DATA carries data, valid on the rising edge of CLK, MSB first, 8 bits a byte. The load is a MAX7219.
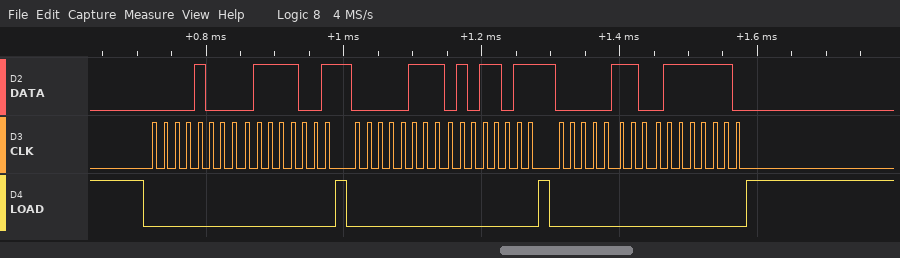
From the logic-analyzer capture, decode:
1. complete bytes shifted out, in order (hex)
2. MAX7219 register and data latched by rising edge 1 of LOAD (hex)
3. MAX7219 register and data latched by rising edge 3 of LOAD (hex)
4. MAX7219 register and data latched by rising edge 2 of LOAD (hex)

0x08 0x79 0x07 0x5B 0x06 0x7E
register 0x8, data 0x79
register 0x6, data 0x7E
register 0x7, data 0x5B
